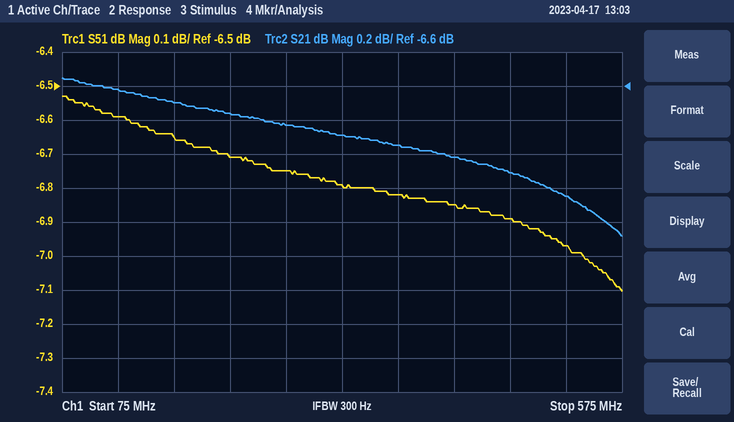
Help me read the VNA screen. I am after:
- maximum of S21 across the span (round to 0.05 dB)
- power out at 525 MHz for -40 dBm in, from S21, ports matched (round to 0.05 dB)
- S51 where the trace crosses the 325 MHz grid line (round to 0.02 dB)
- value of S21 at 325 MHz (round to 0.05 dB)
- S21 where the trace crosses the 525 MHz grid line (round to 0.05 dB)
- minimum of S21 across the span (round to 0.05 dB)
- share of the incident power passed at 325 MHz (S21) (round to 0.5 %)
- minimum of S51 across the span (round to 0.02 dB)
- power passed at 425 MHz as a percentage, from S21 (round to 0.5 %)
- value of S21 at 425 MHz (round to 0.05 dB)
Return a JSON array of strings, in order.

["-6.55 dB", "-47.25 dBm", "-6.80 dB", "-6.90 dB", "-7.25 dB", "-7.50 dB", "20.5 %", "-7.10 dB", "20.0 %", "-7.00 dB"]
